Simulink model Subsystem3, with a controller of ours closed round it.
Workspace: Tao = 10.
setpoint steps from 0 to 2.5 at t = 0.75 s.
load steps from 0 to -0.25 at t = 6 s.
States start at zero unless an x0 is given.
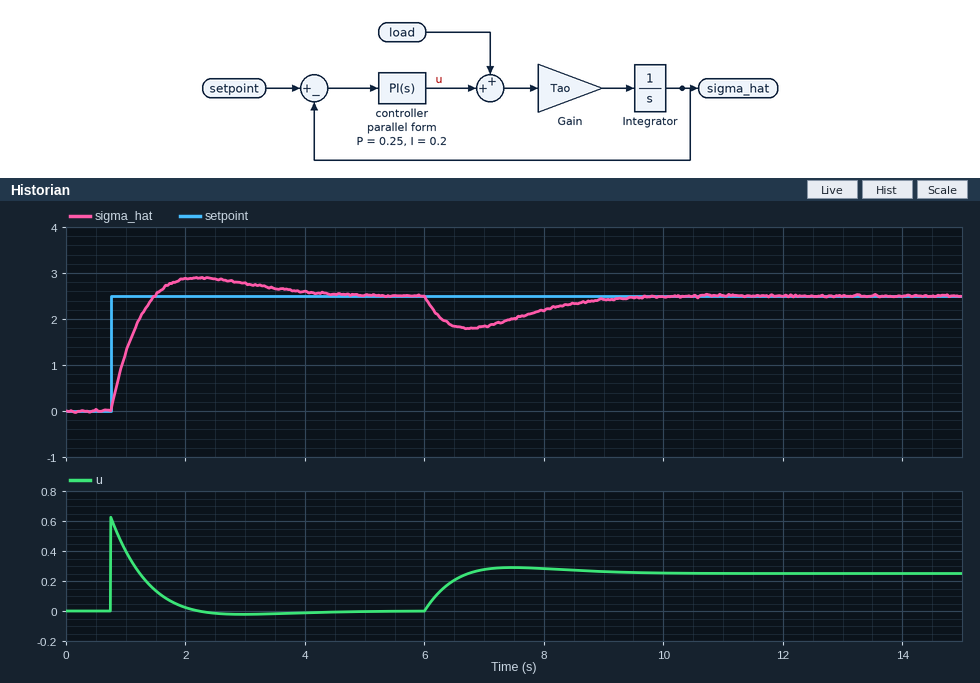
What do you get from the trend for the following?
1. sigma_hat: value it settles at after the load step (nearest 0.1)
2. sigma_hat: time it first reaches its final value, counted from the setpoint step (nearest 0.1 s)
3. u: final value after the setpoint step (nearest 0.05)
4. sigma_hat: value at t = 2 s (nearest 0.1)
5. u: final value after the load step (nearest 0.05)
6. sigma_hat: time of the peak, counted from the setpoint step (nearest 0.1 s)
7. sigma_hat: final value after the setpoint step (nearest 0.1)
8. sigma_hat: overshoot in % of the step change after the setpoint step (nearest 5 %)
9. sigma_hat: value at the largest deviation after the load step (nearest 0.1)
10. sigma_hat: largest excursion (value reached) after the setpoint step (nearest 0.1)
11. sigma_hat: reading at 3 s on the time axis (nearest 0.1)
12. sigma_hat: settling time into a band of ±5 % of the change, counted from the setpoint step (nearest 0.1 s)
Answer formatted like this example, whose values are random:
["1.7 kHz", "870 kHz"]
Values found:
["2.5", "0.7 s", "0.00", "2.9", "0.25", "1.5 s", "2.5", "15 %", "1.8", "2.9", "2.8", "3.0 s"]
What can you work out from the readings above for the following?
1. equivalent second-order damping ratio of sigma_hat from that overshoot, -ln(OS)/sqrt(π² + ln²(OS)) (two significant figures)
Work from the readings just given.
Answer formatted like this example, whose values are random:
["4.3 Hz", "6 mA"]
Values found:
["0.52"]
